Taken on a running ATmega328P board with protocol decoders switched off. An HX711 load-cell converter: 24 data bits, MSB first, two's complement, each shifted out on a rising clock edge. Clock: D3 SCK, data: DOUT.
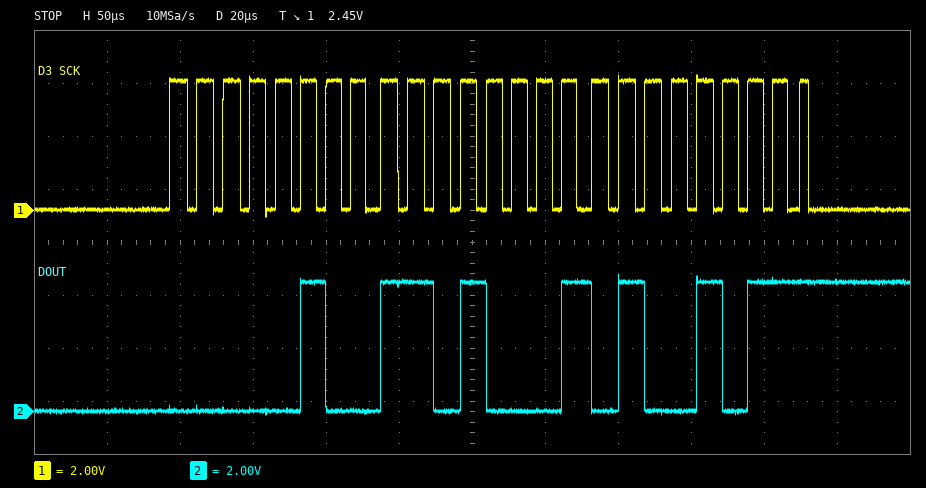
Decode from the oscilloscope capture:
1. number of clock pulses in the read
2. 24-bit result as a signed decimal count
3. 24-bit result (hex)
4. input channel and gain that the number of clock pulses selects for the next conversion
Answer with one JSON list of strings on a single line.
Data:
["25", "315723", "0x04D14B", "channel A, gain 128"]
